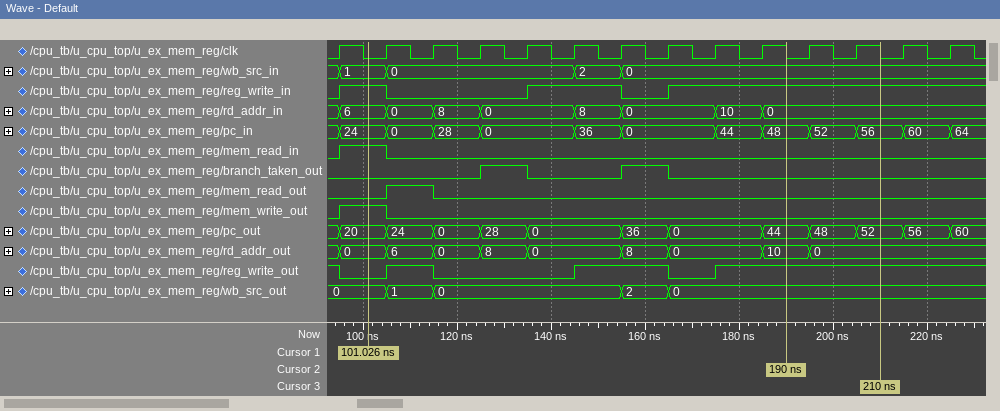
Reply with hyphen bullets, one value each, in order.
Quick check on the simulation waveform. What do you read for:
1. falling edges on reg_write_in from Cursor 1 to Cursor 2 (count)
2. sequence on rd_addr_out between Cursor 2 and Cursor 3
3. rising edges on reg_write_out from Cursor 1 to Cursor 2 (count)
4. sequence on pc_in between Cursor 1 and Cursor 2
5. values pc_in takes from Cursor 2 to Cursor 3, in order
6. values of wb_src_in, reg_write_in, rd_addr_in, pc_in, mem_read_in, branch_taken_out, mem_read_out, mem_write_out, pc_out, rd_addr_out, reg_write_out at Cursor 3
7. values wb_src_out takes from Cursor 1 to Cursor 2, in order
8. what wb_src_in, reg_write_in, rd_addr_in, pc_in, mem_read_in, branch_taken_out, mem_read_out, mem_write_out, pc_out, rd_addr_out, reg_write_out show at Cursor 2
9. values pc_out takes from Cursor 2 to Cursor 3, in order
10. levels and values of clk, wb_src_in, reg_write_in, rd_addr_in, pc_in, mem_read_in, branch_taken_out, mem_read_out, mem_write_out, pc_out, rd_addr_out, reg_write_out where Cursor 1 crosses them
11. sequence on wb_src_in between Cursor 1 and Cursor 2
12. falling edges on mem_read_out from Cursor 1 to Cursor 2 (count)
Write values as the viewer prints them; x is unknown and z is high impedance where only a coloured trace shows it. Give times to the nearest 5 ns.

- 2
- 10, 0
- 3
- 24, 0, 28, 0, 36, 0, 44, 48
- 48, 52, 56
- wb_src_in=0, reg_write_in=1, rd_addr_in=0, pc_in=56, mem_read_in=0, branch_taken_out=0, mem_read_out=0, mem_write_out=0, pc_out=52, rd_addr_out=0, reg_write_out=1
- 0, 1, 0, 2, 0
- wb_src_in=0, reg_write_in=1, rd_addr_in=0, pc_in=48, mem_read_in=0, branch_taken_out=0, mem_read_out=0, mem_write_out=0, pc_out=44, rd_addr_out=10, reg_write_out=1
- 44, 48, 52
- clk=0, wb_src_in=1, reg_write_in=1, rd_addr_in=6, pc_in=24, mem_read_in=1, branch_taken_out=0, mem_read_out=0, mem_write_out=1, pc_out=20, rd_addr_out=0, reg_write_out=0
- 1, 0, 2, 0
- 1
